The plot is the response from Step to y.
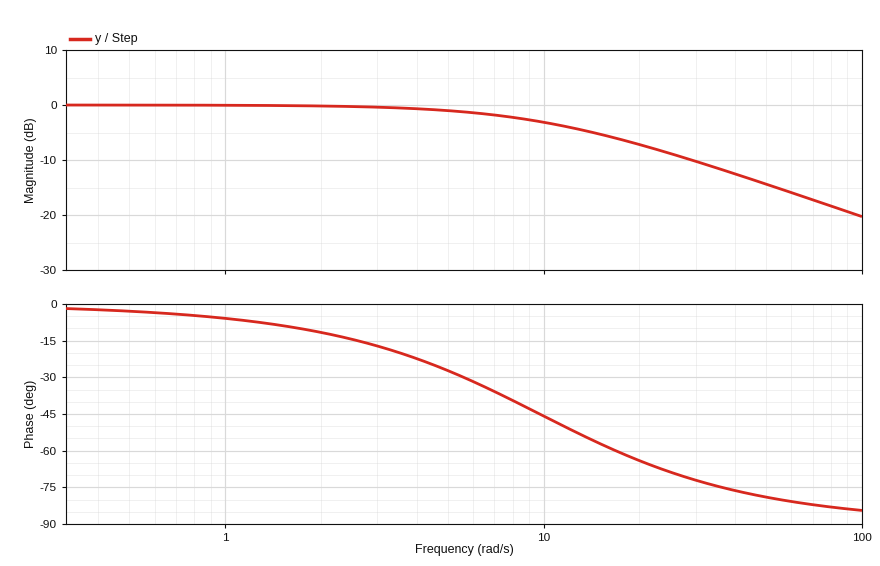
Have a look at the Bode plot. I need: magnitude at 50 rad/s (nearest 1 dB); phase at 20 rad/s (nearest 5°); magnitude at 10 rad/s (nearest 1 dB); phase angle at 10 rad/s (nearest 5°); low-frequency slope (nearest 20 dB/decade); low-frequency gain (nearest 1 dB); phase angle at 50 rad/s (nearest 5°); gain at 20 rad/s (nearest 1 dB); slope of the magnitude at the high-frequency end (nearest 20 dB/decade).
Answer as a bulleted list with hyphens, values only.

- -14 dB
- -65°
- -3 dB
- -45°
- 0 dB/decade
- 0 dB
- -80°
- -7 dB
- -20 dB/decade
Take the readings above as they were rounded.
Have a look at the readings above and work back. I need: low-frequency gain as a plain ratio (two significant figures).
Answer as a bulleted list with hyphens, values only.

- 1.0
